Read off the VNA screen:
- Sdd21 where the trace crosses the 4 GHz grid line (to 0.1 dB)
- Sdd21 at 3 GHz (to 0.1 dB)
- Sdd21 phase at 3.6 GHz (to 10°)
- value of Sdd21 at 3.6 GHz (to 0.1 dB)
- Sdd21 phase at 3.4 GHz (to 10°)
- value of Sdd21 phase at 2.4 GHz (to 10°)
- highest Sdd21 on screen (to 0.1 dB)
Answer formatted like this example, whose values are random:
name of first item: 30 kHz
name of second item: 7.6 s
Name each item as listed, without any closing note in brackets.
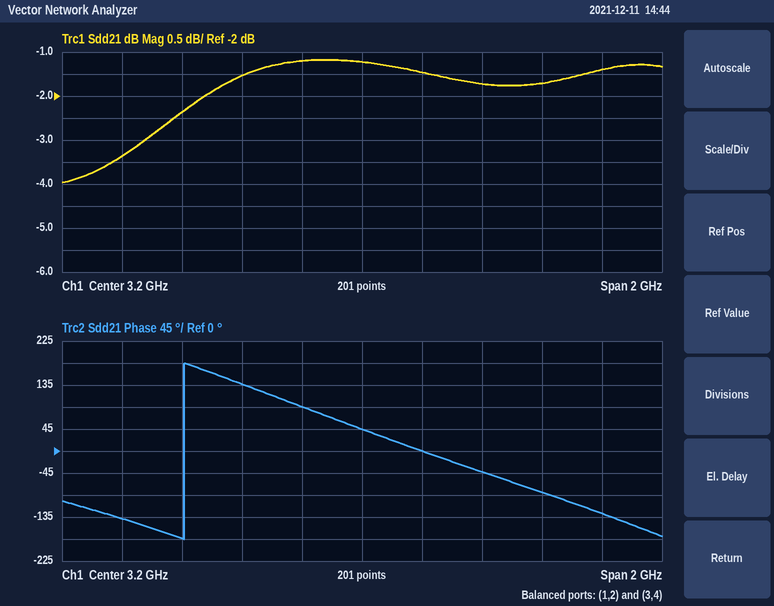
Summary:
Sdd21 where the trace crosses the 4 GHz grid line: -1.4 dB
Sdd21 at 3 GHz: -1.2 dB
Sdd21 phase at 3.6 GHz: -40°
value of Sdd21 at 3.6 GHz: -1.7 dB
Sdd21 phase at 3.4 GHz: 0°
value of Sdd21 phase at 2.4 GHz: -140°
highest Sdd21 on screen: -1.2 dB
